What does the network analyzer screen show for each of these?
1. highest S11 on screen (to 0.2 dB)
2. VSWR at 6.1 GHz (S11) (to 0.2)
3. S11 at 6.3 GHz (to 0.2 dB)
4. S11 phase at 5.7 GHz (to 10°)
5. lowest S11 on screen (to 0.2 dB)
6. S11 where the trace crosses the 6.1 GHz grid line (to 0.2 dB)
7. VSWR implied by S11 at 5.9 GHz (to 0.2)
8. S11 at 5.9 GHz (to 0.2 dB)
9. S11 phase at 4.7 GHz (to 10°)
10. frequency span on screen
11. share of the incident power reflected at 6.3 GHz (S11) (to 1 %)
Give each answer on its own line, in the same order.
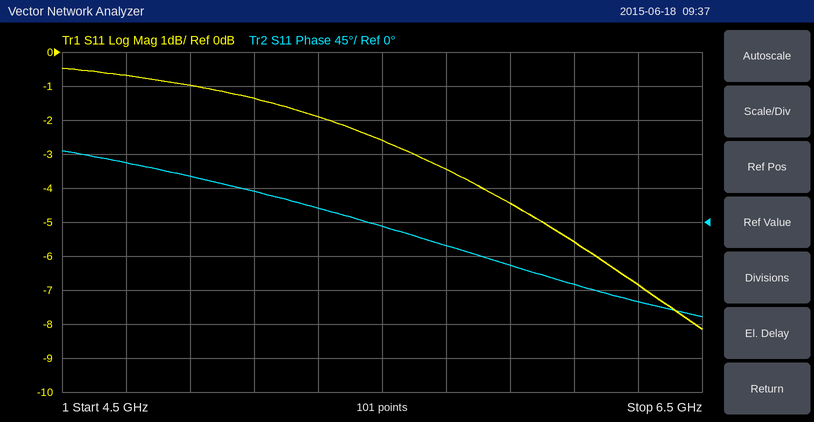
-0.4 dB
3.2
-6.8 dB
-30°
-8.2 dB
-5.6 dB
4.0
-4.4 dB
80°
2 GHz
21 %
